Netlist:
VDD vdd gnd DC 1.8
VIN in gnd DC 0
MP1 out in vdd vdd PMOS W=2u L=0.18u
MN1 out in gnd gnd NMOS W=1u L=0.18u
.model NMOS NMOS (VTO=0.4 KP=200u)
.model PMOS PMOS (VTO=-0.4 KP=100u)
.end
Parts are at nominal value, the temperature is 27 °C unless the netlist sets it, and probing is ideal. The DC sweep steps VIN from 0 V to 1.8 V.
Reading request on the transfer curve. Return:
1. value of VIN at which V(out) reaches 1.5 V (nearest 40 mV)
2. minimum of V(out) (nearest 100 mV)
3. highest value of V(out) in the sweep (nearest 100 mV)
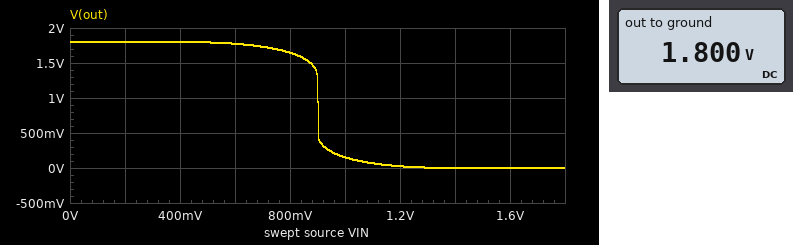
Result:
880 mV
0 V
1.8 V
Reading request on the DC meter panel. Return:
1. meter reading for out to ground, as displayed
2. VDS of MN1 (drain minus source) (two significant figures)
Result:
1.800 V
1.8 V
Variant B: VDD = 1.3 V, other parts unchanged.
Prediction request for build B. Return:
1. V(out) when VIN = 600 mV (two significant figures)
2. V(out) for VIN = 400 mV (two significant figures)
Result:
1.2 V
1.3 V
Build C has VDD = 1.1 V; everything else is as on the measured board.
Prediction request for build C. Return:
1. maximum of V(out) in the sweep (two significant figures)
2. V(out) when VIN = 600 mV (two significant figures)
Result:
1.1 V
27 mV
